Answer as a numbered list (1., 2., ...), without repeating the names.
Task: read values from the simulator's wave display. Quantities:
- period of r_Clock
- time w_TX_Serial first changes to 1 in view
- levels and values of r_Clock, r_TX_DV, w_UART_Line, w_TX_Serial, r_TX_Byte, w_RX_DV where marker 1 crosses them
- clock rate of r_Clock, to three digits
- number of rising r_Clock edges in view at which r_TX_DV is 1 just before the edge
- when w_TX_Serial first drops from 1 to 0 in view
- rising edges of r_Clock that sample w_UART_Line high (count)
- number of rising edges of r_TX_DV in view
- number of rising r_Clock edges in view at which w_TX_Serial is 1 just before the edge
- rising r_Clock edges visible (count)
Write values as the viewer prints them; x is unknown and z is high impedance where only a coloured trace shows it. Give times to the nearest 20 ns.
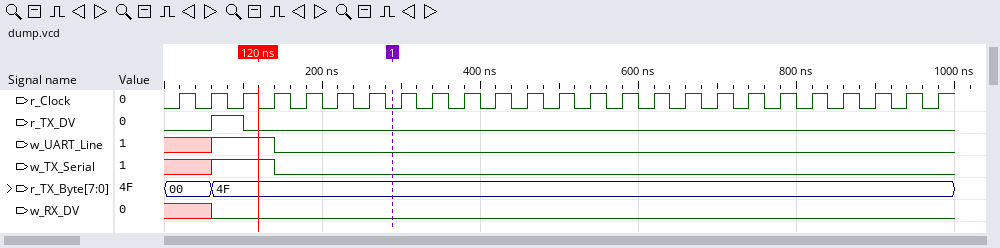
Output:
1. 40 ns
2. 60 ns
3. r_Clock=0, r_TX_DV=0, w_UART_Line=0, w_TX_Serial=0, r_TX_Byte=4F, w_RX_DV=0
4. 25.0 MHz
5. 1
6. 140 ns
7. 2
8. 1
9. 2
10. 25
